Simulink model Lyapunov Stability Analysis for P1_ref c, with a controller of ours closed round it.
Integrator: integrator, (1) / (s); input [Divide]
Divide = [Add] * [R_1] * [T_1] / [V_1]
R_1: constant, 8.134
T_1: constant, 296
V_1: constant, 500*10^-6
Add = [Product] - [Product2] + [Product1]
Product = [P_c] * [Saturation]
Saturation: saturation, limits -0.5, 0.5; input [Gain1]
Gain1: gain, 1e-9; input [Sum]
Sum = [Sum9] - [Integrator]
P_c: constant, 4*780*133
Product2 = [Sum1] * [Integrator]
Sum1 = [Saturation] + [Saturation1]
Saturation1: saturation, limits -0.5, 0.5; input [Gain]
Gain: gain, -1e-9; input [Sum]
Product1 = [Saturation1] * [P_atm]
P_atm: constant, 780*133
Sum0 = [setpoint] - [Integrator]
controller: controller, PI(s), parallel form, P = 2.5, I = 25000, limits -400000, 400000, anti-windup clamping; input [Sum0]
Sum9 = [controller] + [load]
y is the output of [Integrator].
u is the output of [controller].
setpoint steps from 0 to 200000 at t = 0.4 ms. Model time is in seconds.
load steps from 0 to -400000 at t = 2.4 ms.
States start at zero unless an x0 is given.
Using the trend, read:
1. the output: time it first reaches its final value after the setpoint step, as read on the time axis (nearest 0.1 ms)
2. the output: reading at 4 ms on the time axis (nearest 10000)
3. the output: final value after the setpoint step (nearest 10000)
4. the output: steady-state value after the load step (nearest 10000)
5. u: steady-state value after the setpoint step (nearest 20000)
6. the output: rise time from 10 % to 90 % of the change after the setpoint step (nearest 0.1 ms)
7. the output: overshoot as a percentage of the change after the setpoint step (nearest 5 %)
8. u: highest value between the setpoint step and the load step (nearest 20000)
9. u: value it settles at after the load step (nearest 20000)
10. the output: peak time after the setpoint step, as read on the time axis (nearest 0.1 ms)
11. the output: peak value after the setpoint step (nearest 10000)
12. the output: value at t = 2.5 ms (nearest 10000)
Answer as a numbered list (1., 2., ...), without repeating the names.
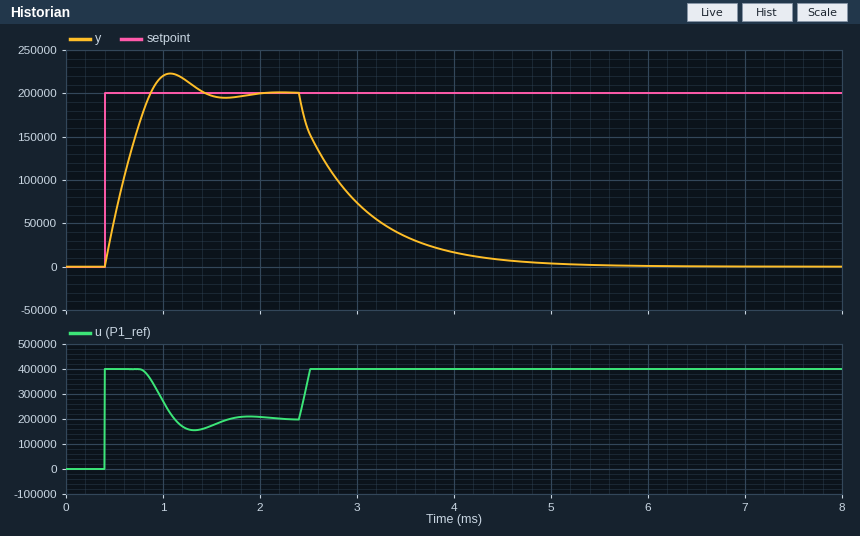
1. 0.9 ms
2. 20000
3. 200000
4. 0
5. 200000
6. 0.4 ms
7. 10 %
8. 400000
9. 400000
10. 1.1 ms
11. 220000
12. 160000
